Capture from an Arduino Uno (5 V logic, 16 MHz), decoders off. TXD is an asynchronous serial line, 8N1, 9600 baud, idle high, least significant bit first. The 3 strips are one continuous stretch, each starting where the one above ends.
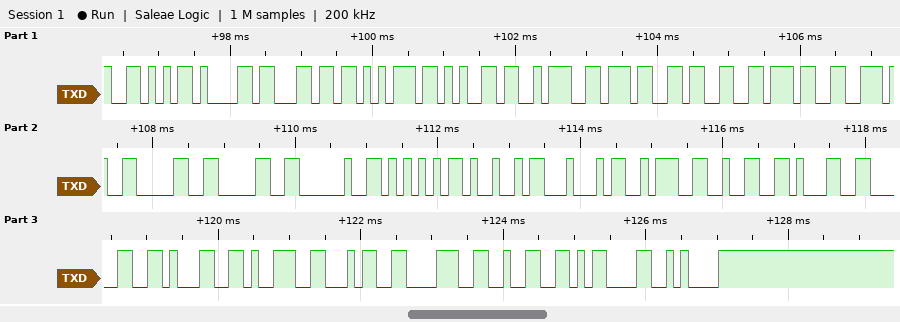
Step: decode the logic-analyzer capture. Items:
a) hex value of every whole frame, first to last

56 61 6C 75 65 3A 37 33 37 2E 30 30 20 55 49 44 3A 32 31 30 31 39 34 38 32 0D 0A
